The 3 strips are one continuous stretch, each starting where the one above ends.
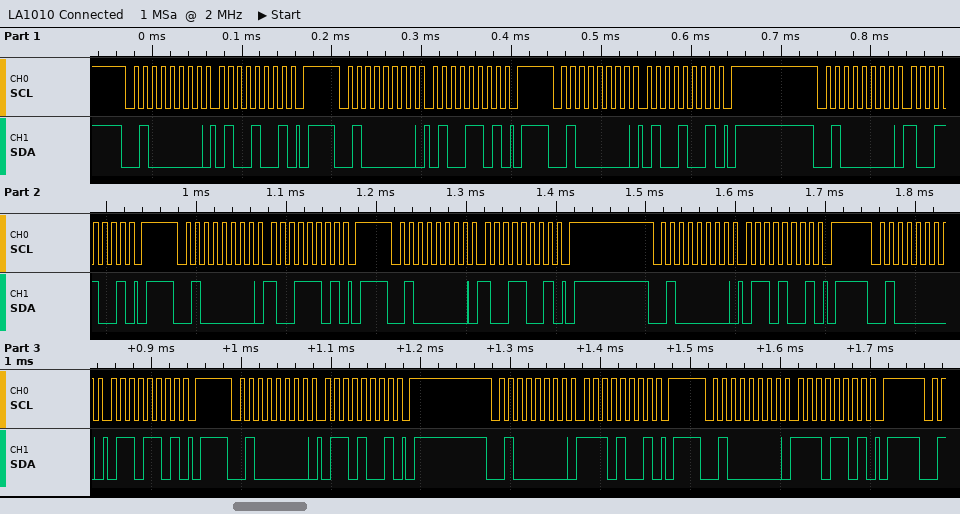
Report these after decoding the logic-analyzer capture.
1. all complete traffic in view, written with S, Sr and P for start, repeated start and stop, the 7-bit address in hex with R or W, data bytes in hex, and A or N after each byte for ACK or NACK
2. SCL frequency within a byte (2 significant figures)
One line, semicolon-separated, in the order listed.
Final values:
S 20W A 49 A P S 20W A 4D A P S 20W A 49 A P S 20W A 99 A P S 20W A 9D A P S 20W A 99 A P S 20W A 69 A P S 20W A 6D A P S 20W A 69 A P S 20W A E9 A P S 20W A ED A P; 100 kHz
